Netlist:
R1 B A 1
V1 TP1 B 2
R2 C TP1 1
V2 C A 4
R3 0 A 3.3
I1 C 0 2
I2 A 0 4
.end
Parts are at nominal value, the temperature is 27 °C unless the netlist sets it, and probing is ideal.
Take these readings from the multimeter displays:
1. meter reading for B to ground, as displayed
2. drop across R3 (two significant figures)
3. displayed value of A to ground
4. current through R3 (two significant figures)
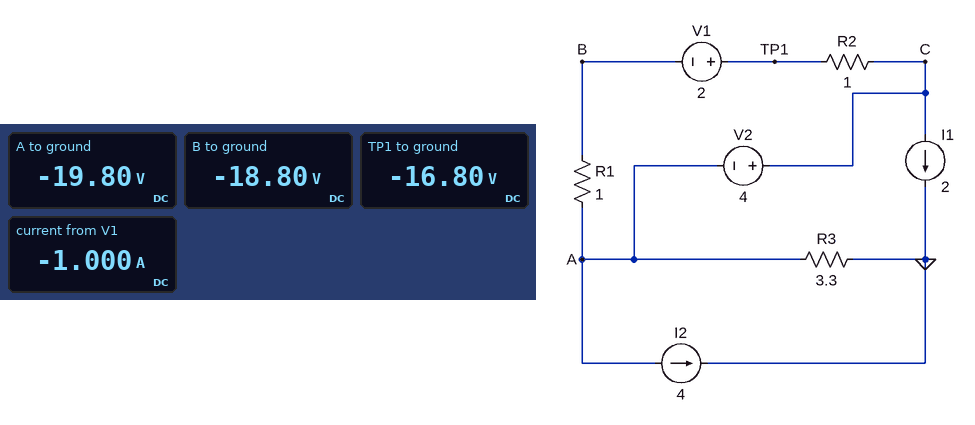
-18.80 V
20 V
-19.80 V
6.0 A
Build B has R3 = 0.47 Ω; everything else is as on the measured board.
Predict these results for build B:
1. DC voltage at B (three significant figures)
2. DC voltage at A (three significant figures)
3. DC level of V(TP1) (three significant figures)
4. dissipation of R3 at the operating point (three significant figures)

-1.82 V
-2.82 V
180 mV
16.9 W
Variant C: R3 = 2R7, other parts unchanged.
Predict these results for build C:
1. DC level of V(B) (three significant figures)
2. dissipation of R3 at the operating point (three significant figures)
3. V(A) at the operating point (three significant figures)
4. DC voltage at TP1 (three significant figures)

-15.2 V
97.2 W
-16.2 V
-13.2 V
